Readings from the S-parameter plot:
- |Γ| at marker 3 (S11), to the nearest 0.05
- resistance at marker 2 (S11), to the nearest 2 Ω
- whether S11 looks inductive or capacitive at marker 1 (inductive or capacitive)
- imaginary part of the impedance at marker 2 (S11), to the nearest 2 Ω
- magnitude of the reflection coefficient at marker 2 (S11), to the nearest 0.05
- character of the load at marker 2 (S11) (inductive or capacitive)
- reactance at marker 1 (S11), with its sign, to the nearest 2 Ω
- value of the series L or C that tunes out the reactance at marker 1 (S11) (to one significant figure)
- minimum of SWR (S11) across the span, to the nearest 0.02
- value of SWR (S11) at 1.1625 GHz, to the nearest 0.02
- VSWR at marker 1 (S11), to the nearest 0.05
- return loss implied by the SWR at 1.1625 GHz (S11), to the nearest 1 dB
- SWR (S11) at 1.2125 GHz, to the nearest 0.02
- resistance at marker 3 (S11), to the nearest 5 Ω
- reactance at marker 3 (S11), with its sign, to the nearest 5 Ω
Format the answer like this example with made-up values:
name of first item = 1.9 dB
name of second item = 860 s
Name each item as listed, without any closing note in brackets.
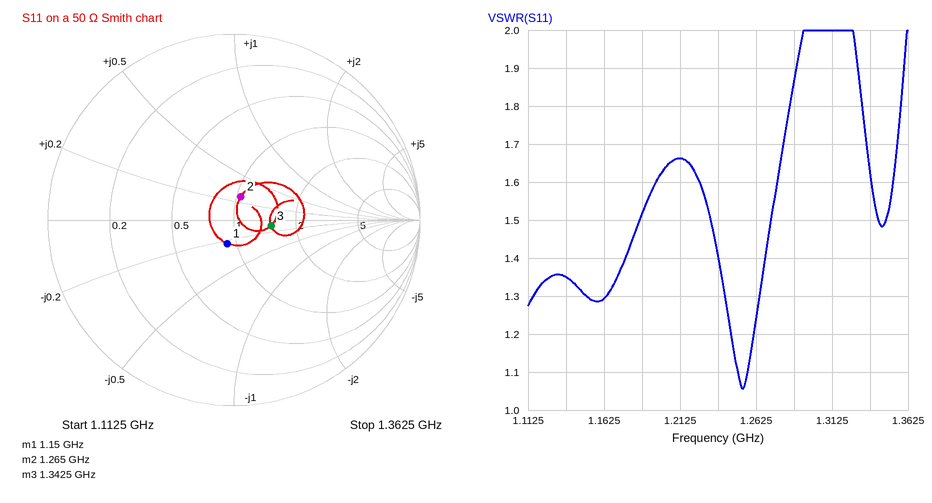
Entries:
|Γ| at marker 3 (S11), to the nearest 0.05 = 0.20
resistance at marker 2 (S11), to the nearest 2 Ω = 52 Ω
whether S11 looks inductive or capacitive at marker 1 = capacitive
imaginary part of the impedance at marker 2 (S11), to the nearest 2 Ω = +14 Ω
magnitude of the reflection coefficient at marker 2 (S11), to the nearest 0.05 = 0.15
character of the load at marker 2 (S11) = inductive
reactance at marker 1 (S11), with its sign, to the nearest 2 Ω = -12 Ω
value of the series L or C that tunes out the reactance at marker 1 (S11) = 2 nH
minimum of SWR (S11) across the span, to the nearest 0.02 = 1.06
value of SWR (S11) at 1.1625 GHz, to the nearest 0.02 = 1.30
VSWR at marker 1 (S11), to the nearest 0.05 = 1.30
return loss implied by the SWR at 1.1625 GHz (S11), to the nearest 1 dB = 18 dB
SWR (S11) at 1.2125 GHz, to the nearest 0.02 = 1.66
resistance at marker 3 (S11), to the nearest 5 Ω = 75 Ω
reactance at marker 3 (S11), with its sign, to the nearest 5 Ω = -5 Ω
